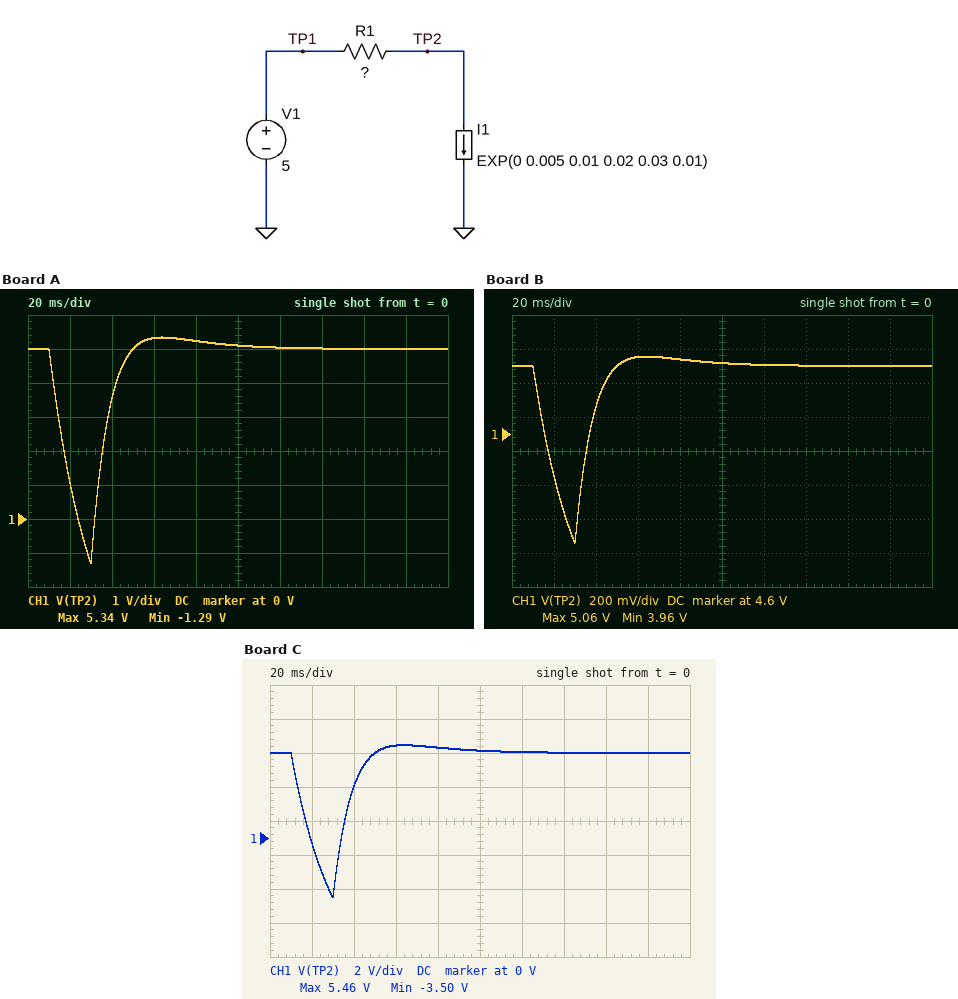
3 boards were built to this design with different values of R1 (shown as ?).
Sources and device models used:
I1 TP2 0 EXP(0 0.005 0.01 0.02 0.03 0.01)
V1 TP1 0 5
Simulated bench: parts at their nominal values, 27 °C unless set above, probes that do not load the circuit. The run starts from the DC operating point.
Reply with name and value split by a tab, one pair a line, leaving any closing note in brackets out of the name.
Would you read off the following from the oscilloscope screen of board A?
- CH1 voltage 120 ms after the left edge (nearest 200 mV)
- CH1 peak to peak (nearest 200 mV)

CH1 voltage 120 ms after the left edge	5.0 V
CH1 peak to peak	6.6 V
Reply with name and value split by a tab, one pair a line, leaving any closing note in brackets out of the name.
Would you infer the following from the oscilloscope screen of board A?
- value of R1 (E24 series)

value of R1	2 kΩ
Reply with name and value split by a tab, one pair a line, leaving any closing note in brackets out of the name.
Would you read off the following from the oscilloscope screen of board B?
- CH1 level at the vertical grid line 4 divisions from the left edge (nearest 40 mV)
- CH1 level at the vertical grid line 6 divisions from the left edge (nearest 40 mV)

CH1 level at the vertical grid line 4 divisions from the left edge	5.04 V
CH1 level at the vertical grid line 6 divisions from the left edge	5.00 V
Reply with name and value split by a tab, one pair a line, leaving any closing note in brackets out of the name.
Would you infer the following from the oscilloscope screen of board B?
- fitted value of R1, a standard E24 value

fitted value of R1, a standard E24 value	330 Ω
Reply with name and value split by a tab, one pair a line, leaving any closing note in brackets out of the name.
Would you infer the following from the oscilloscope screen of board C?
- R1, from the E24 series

R1, from the E24 series	2.7 kΩ
